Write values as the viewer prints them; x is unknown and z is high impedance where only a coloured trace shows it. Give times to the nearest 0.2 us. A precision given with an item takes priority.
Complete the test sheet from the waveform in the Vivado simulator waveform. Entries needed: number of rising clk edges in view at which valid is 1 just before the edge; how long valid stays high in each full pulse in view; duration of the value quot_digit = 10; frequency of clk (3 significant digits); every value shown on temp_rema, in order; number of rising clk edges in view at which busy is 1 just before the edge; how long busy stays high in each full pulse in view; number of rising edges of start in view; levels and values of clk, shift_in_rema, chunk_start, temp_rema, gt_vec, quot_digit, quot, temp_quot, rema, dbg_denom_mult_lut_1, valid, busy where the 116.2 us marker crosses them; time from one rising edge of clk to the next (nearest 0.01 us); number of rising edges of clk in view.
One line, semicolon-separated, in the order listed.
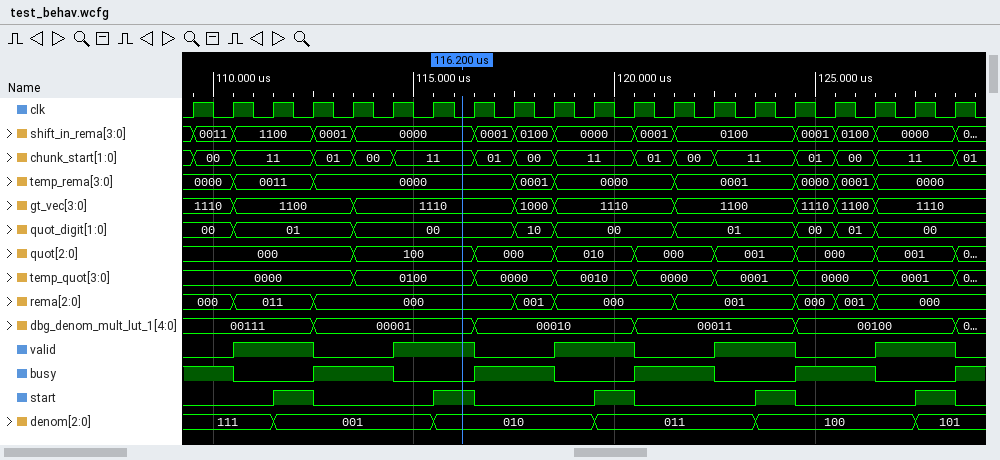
10; 2 us, 2 us, 2 us, 2 us, 2 us; 1 us; 1.00 MHz; 0000, 0011, 0000, 0001, 0000, 0001, 0000, 0001, 0000; 10; 2 us, 2 us, 2 us, 2 us; 5; clk=0, shift_in_rema=0000, chunk_start=11, temp_rema=0000, gt_vec=1110, quot_digit=00, quot=100, temp_quot=0100, rema=000, dbg_denom_mult_lut_1=00001, valid=1, busy=0; 1 us; 20
